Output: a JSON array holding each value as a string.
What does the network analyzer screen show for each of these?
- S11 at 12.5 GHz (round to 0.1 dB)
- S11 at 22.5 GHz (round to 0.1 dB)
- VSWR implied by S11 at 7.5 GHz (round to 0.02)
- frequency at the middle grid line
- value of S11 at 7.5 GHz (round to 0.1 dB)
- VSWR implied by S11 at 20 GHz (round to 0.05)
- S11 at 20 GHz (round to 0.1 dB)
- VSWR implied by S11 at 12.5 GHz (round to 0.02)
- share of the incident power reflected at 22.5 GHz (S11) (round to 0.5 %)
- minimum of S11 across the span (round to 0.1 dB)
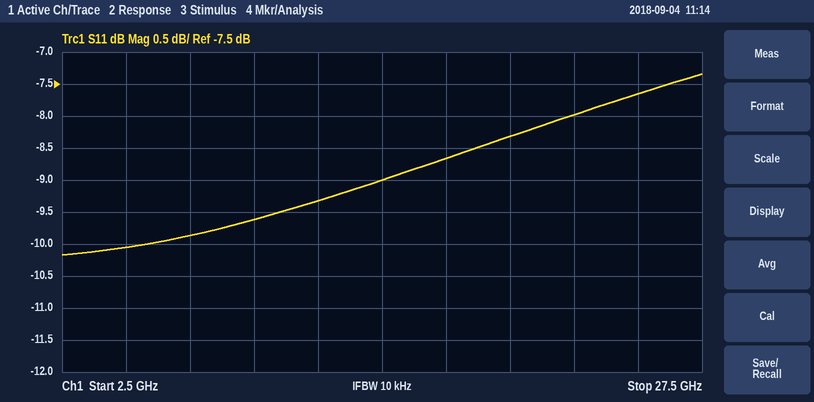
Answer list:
["-9.3 dB", "-8.0 dB", "1.94", "15 GHz", "-9.9 dB", "2.25", "-8.3 dB", "2.04", "16.0 %", "-10.2 dB"]
